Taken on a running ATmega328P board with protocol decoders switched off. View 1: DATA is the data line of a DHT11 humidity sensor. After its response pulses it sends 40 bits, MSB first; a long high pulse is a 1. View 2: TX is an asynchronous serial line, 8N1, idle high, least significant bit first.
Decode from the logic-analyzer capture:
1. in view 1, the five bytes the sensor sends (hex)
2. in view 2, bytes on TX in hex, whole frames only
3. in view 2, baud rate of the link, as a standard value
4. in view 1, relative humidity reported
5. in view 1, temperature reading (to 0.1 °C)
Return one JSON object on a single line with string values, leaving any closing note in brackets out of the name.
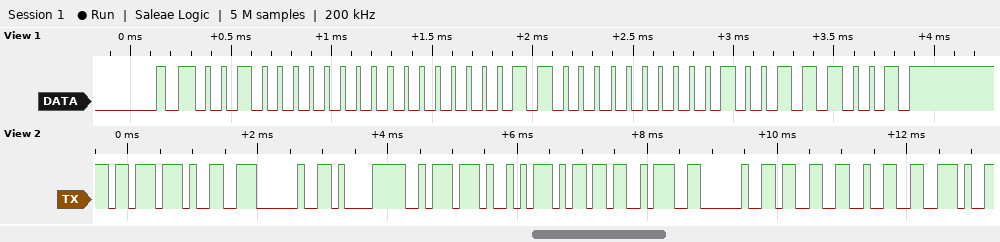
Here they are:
{"in view 1, the five bytes the sensor sends": "20 00 18 01 39", "in view 2, bytes on TX in hex, whole frames only": "BB 99 20 E1 BA A9 6D 3A 20 33 32 2E", "in view 2, baud rate of the link, as a standard value": "9600 baud", "in view 1, relative humidity reported": "32 %", "in view 1, temperature reading": "24.1 °C"}
